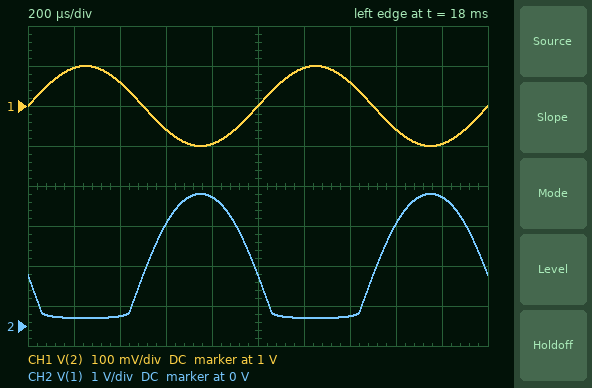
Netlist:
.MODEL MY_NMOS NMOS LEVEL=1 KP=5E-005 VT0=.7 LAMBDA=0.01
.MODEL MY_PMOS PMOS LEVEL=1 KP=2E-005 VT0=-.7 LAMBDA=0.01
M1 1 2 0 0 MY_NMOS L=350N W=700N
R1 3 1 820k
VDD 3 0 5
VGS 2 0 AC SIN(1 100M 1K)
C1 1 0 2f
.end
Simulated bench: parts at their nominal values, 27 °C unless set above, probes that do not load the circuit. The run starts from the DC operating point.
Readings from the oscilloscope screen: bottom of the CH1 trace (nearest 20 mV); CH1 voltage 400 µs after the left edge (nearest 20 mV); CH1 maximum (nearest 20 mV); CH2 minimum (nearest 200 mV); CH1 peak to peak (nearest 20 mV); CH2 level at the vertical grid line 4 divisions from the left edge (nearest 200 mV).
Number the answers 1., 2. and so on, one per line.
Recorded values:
1. 900 mV
2. 1.06 V
3. 1.10 V
4. 200 mV
5. 200 mV
6. 3.2 V
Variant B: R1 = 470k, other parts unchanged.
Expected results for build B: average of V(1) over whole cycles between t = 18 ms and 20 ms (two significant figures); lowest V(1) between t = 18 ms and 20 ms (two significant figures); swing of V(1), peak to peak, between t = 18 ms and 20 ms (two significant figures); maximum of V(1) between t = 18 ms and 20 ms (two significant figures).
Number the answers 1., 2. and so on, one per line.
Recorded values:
1. 2.7 V
2. 1.2 V
3. 2.8 V
4. 4.0 V
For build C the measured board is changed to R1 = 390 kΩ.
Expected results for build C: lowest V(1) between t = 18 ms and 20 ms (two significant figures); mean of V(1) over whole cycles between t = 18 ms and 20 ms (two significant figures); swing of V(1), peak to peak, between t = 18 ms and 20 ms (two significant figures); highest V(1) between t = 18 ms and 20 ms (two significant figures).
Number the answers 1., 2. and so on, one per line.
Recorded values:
1. 1.8 V
2. 3.1 V
3. 2.4 V
4. 4.2 V
